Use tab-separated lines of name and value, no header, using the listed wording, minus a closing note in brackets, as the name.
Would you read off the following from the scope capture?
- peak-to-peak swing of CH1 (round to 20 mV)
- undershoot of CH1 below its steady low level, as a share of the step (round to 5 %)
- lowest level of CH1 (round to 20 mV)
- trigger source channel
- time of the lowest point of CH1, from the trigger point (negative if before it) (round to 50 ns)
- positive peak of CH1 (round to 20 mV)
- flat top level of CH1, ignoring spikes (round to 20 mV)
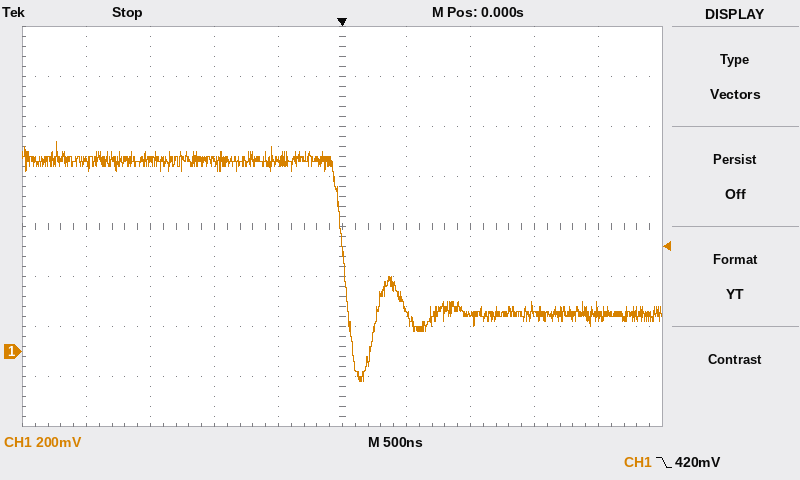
peak-to-peak swing of CH1	960 mV
undershoot of CH1 below its steady low level, as a share of the step	45 %
lowest level of CH1	-120 mV
trigger source channel	CH1
time of the lowest point of CH1, from the trigger point (negative if before it)	+150 ns
positive peak of CH1	840 mV
flat top level of CH1, ignoring spikes	760 mV
